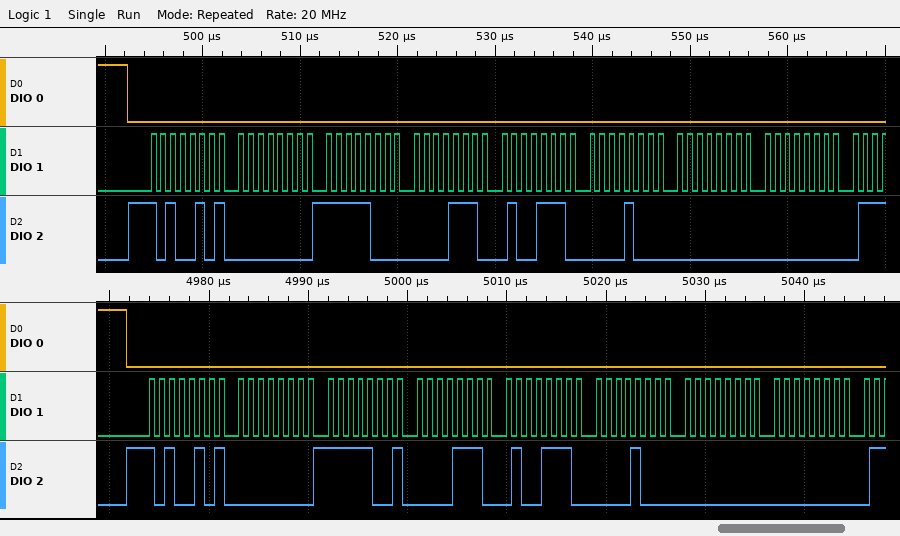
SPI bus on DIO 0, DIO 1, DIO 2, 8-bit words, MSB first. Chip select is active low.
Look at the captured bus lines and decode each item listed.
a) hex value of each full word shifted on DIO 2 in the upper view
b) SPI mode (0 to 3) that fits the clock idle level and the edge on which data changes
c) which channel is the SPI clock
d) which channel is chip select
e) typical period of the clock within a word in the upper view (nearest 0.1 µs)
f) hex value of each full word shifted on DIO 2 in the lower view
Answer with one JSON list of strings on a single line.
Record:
["A5, 00, F8, 0E, 4E, 08, 00, 00", "0", "DIO 1", "DIO 0", "1 µs", "A5, 00, F9, 0E, 4E, 08, 00, 00"]
